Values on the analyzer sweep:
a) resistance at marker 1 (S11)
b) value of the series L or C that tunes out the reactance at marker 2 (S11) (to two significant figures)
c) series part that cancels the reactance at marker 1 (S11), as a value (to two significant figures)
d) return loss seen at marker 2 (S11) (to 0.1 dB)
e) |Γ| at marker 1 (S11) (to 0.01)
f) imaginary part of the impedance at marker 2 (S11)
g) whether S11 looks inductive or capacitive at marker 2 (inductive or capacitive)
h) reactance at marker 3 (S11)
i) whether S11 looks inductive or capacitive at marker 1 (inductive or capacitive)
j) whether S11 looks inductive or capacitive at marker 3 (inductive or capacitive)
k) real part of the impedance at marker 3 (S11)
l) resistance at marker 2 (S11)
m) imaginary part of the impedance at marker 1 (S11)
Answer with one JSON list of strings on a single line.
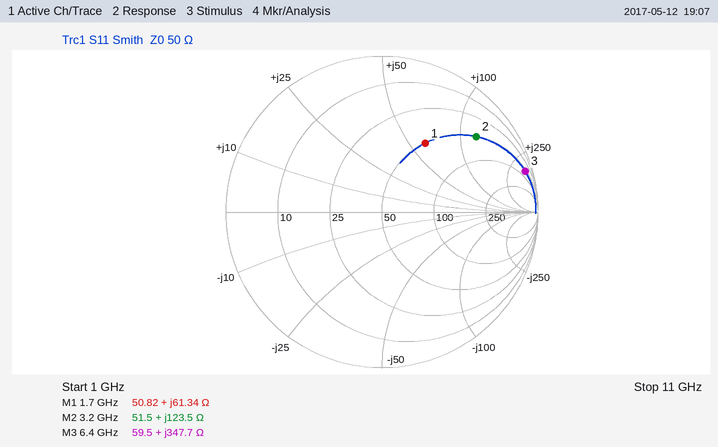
["50.82 Ω", "400 fF", "1.5 pF", "2.2 dB", "0.52", "+123.5 Ω", "inductive", "+347.7 Ω", "inductive", "inductive", "59.5 Ω", "51.5 Ω", "+61.34 Ω"]
